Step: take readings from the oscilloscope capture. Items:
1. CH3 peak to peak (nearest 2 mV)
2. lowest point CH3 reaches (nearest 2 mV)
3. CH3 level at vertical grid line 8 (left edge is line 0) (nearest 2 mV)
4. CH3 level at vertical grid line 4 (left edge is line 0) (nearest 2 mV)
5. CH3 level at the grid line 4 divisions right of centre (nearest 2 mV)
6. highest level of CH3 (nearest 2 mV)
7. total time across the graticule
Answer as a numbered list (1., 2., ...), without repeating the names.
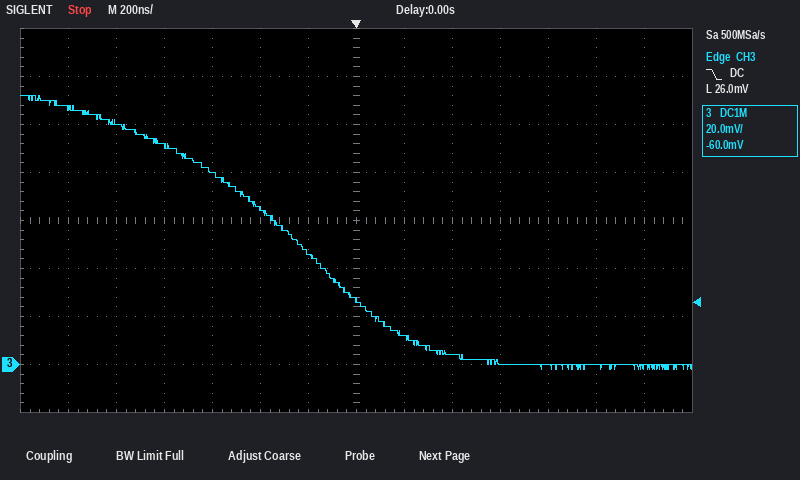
1. 114 mV
2. -2 mV
3. 12 mV
4. 80 mV
5. 0 mV
6. 112 mV
7. 2.8 µs
